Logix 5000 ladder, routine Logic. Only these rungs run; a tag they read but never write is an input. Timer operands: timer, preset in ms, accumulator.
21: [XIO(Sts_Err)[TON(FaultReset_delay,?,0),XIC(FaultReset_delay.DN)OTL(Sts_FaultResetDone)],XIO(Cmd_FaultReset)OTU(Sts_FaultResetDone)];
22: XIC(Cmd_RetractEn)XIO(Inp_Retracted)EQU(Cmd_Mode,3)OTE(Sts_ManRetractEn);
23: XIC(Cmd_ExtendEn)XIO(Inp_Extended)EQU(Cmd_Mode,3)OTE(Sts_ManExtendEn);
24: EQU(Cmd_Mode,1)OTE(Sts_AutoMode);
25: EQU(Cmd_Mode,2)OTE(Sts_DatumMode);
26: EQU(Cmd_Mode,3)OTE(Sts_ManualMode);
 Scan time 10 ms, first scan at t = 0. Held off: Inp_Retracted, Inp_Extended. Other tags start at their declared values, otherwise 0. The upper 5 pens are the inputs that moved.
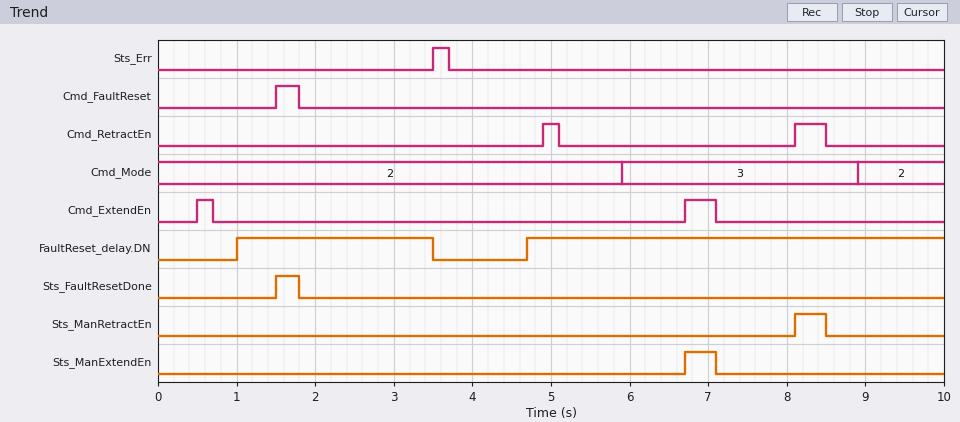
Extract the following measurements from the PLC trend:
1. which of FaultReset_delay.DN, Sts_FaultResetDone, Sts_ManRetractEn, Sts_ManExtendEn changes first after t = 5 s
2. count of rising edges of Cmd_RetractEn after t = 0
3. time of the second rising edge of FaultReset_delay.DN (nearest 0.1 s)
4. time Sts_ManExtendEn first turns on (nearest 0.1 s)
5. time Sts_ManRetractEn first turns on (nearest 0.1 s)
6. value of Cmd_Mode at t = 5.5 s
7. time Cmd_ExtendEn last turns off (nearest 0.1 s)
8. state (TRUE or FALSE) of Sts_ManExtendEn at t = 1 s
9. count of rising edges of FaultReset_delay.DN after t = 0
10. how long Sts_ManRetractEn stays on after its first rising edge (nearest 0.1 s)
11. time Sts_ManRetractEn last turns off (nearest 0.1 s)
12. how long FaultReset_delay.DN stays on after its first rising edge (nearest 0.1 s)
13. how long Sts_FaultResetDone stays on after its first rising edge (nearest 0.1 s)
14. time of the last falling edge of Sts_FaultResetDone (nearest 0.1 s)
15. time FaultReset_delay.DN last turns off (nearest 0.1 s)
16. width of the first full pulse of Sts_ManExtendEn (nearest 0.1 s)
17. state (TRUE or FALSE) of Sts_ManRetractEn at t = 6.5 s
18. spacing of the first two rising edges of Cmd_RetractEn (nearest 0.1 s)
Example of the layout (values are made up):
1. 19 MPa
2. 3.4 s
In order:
1. Sts_ManExtendEn
2. 2
3. 4.7 s
4. 6.7 s
5. 8.1 s
6. 2
7. 7.1 s
8. FALSE
9. 2
10. 0.4 s
11. 8.5 s
12. 2.5 s
13. 0.3 s
14. 1.8 s
15. 3.5 s
16. 0.4 s
17. FALSE
18. 3.2 s
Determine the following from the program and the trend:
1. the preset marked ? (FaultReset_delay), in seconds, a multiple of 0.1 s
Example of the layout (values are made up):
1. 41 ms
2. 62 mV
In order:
1. 1.0 s
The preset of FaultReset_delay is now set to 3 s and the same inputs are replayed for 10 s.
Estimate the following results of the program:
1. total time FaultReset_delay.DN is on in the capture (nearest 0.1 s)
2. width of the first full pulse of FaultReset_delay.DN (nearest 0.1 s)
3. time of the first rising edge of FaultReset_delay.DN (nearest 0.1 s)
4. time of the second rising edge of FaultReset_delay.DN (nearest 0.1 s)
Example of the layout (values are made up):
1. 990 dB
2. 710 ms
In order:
1. 3.8 s
2. 0.5 s
3. 3.0 s
4. 6.7 s
